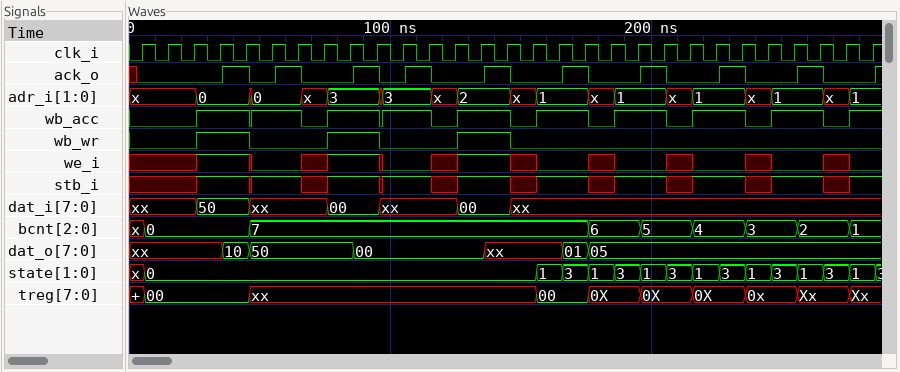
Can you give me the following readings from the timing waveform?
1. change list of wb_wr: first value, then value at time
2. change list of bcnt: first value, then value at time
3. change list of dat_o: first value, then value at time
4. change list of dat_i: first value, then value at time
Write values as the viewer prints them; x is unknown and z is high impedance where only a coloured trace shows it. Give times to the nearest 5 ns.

0, 1 at 25 ns, 0 at 45 ns, 1 at 75 ns, 0 at 95 ns, 1 at 125 ns, 0 at 145 ns
x, 0 at 5 ns, 7 at 45 ns, 6 at 175 ns, 5 at 195 ns, 4 at 215 ns, 3 at 235 ns, 2 at 255 ns, 1 at 275 ns
xx, 10 at 35 ns, 50 at 45 ns, 00 at 85 ns, xx at 135 ns, 01 at 165 ns, 05 at 175 ns
xx, 50 at 25 ns, xx at 45 ns, 00 at 75 ns, xx at 95 ns, 00 at 125 ns, xx at 145 ns
